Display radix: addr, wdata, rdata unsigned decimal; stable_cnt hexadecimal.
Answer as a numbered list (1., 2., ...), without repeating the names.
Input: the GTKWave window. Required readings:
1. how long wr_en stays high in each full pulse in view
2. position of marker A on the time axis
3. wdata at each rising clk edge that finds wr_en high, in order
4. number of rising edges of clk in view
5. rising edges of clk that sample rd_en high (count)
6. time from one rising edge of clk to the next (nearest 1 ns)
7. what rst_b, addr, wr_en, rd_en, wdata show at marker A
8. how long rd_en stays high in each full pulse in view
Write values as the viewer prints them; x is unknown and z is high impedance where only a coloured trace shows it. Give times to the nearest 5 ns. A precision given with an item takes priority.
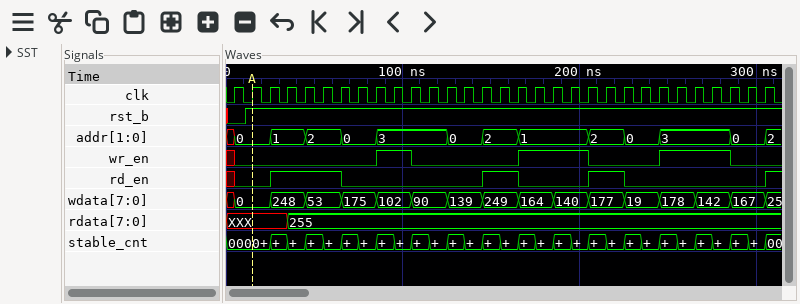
1. 20 ns, 40 ns, 40 ns
2. 15 ns
3. 102, 102, 164, 164, 140, 140, 178, 178, 142, 142
4. 31
5. 8
6. 10 ns
7. rst_b=1, addr=0, wr_en=0, rd_en=0, wdata=0
8. 40 ns, 20 ns, 20 ns
